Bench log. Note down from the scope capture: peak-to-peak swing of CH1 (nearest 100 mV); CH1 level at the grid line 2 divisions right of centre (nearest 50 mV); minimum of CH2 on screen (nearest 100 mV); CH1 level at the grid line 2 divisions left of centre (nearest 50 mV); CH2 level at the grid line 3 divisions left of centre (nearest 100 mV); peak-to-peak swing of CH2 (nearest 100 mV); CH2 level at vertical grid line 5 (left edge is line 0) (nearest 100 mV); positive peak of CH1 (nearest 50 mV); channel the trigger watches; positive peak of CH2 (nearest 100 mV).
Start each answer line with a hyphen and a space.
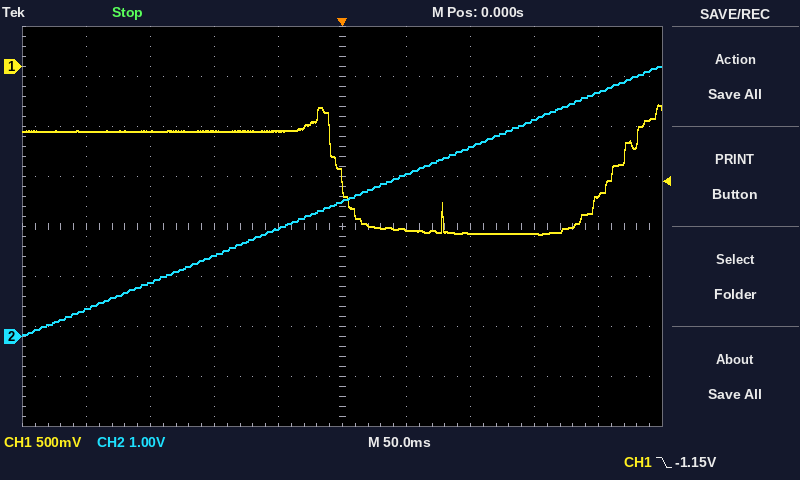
- 1.30 V
- -1.65 V
- 0.0 V
- -650 mV
- 1.1 V
- 5.4 V
- 2.7 V
- -400 mV
- CH1
- 5.4 V
